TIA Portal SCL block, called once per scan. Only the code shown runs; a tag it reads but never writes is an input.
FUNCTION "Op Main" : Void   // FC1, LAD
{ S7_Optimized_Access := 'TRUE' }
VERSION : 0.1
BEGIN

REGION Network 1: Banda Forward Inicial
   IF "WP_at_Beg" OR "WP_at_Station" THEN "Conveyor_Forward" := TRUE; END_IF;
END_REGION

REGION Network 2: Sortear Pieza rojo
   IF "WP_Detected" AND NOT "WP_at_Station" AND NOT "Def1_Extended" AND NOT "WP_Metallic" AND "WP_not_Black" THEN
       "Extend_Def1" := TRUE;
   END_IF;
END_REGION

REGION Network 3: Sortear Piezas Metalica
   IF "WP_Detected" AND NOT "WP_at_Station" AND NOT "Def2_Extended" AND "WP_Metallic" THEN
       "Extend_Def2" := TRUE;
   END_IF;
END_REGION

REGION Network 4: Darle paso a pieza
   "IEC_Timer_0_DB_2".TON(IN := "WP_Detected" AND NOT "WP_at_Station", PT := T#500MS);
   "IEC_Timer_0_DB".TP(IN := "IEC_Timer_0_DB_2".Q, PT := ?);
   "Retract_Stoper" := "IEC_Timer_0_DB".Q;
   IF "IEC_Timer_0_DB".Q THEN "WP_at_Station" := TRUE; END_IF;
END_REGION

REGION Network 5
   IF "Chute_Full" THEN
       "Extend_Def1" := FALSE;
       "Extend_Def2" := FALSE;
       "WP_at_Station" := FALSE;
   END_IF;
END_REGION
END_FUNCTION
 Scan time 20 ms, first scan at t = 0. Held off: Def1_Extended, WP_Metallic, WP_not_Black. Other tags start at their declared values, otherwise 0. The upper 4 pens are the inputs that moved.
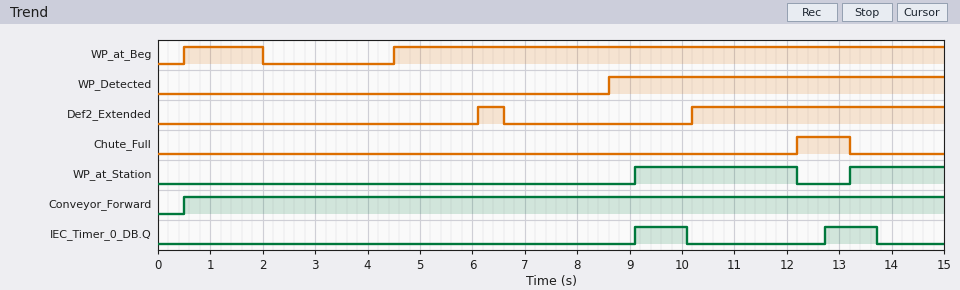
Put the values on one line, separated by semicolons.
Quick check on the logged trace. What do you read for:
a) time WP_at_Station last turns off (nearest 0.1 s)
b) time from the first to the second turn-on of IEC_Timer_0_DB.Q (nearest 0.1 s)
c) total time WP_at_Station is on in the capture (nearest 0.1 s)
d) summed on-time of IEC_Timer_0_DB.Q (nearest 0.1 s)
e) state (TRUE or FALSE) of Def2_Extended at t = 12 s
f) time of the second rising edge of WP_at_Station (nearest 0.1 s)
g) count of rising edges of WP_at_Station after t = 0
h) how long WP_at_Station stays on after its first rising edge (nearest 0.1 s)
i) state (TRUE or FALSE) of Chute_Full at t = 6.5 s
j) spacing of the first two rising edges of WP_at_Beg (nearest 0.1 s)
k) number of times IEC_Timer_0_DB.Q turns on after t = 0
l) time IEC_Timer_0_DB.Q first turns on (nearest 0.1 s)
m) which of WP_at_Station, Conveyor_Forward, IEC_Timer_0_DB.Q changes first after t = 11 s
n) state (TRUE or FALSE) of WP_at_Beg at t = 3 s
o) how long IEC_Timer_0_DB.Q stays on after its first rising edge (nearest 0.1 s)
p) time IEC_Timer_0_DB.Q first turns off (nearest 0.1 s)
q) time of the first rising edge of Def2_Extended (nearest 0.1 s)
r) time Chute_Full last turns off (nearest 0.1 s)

12.2 s; 3.6 s; 4.9 s; 2.0 s; TRUE; 13.2 s; 2; 3.1 s; FALSE; 4.0 s; 2; 9.1 s; WP_at_Station; FALSE; 1.0 s; 10.1 s; 6.1 s; 13.2 s
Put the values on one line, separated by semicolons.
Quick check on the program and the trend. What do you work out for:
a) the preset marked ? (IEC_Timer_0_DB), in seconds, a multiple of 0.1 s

1.0 s
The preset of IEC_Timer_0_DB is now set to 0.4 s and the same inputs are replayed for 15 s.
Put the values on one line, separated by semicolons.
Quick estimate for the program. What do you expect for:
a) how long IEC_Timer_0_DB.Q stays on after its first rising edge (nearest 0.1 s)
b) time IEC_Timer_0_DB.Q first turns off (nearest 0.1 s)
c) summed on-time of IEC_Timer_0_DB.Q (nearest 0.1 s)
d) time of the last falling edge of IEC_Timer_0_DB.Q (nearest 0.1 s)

0.4 s; 9.5 s; 0.8 s; 13.1 s
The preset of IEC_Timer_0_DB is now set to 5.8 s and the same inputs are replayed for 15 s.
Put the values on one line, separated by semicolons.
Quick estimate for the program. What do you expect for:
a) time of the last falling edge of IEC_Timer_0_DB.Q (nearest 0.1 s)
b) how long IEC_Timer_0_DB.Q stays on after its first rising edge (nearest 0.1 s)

14.9 s; 5.8 s
